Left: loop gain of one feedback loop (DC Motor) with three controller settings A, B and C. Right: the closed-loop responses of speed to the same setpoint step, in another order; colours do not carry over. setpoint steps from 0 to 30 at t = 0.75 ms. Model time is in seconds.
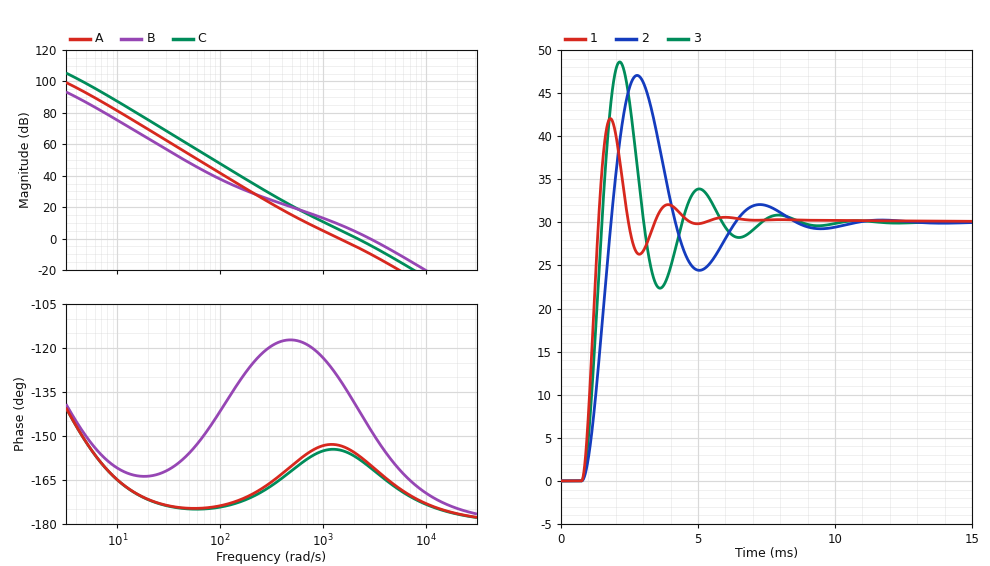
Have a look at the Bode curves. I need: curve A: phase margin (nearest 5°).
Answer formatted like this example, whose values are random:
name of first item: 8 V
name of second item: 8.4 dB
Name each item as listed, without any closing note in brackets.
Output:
curve A: phase margin: 25°
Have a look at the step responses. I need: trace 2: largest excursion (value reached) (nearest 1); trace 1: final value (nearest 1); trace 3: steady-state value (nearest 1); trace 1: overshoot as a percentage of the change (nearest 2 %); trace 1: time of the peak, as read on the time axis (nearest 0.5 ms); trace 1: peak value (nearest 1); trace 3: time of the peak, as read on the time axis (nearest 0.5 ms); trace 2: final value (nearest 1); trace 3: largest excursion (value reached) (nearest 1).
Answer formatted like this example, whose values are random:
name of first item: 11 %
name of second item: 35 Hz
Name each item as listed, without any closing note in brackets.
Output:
trace 2: largest excursion (value reached): 47
trace 1: final value: 30
trace 3: steady-state value: 30
trace 1: overshoot as a percentage of the change: 40 %
trace 1: time of the peak, as read on the time axis: 2.0 ms
trace 1: peak value: 42
trace 3: time of the peak, as read on the time axis: 2.0 ms
trace 2: final value: 30
trace 3: largest excursion (value reached): 49
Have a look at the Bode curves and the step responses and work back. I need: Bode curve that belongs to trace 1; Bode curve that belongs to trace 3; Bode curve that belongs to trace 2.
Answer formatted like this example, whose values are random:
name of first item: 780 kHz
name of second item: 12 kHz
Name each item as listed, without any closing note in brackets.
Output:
Bode curve that belongs to trace 1: B
Bode curve that belongs to trace 3: C
Bode curve that belongs to trace 2: A
